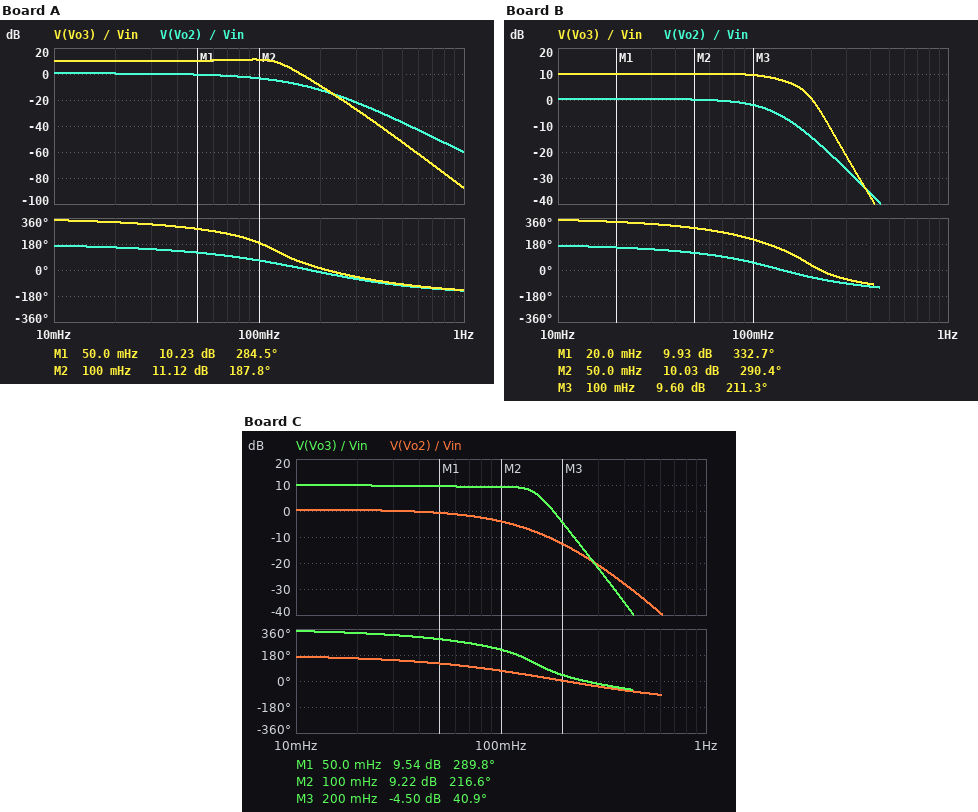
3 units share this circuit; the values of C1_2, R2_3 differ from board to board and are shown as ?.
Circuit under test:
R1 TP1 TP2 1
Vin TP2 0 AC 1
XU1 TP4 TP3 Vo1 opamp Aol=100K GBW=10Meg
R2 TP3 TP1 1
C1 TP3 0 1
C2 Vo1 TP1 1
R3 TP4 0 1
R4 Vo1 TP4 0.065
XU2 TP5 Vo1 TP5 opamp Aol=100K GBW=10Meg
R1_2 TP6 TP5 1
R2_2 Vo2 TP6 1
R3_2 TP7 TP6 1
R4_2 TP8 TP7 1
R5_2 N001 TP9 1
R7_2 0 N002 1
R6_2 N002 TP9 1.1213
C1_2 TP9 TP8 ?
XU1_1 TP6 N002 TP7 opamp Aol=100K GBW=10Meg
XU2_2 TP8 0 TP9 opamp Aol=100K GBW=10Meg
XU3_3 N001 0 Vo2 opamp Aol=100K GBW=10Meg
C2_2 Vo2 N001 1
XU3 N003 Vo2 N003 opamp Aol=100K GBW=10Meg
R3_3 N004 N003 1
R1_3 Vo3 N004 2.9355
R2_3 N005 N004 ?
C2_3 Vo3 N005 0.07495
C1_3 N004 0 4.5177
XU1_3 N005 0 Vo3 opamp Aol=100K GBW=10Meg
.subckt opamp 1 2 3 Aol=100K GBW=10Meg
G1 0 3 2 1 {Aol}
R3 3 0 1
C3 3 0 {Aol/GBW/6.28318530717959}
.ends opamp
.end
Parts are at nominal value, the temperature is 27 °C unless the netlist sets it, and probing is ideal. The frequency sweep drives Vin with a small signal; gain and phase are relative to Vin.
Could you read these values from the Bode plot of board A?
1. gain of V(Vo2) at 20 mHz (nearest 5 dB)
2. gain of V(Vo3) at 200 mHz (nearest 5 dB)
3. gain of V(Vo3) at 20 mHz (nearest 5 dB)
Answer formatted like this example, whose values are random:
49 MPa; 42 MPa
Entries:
0 dB; -10 dB; 10 dB
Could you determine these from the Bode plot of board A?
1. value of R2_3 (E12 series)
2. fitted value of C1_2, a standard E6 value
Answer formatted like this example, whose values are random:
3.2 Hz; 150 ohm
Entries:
1.8 Ω; 680 mF
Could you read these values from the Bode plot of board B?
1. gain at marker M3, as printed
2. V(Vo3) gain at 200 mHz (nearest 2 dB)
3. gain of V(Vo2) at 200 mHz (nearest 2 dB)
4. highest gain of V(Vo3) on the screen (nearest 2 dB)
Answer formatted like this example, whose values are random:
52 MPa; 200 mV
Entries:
9.60 dB; 0 dB; -14 dB; 10 dB
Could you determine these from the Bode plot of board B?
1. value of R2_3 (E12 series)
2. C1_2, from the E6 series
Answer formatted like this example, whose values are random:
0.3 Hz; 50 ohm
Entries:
0.68 Ω; 1.5 F
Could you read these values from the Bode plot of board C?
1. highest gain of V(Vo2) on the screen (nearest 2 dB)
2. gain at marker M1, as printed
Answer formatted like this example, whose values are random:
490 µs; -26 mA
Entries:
0 dB; 9.54 dB
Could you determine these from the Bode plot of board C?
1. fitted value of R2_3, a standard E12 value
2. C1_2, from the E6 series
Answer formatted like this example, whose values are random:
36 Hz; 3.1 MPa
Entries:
1.2 Ω; 330 mF
